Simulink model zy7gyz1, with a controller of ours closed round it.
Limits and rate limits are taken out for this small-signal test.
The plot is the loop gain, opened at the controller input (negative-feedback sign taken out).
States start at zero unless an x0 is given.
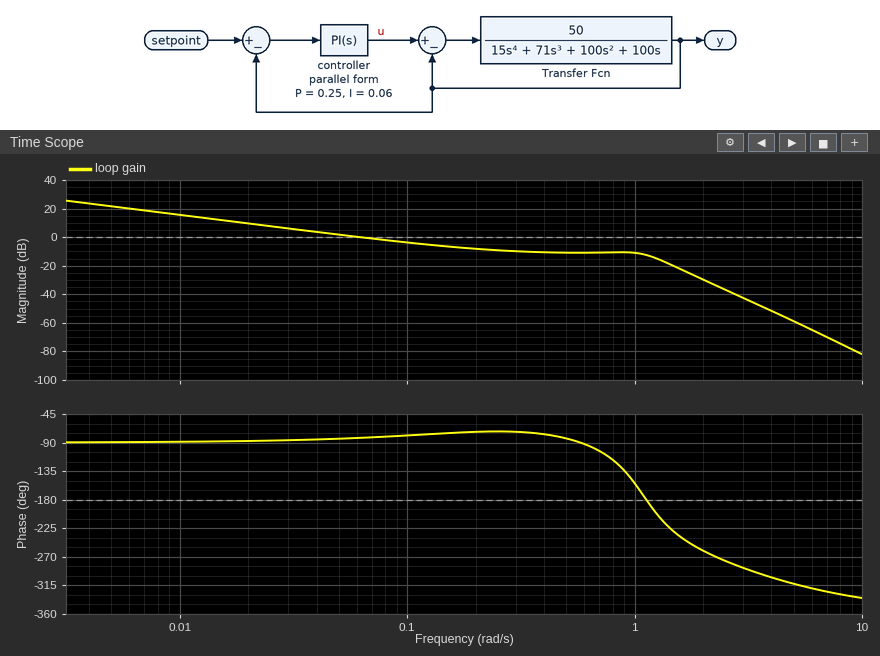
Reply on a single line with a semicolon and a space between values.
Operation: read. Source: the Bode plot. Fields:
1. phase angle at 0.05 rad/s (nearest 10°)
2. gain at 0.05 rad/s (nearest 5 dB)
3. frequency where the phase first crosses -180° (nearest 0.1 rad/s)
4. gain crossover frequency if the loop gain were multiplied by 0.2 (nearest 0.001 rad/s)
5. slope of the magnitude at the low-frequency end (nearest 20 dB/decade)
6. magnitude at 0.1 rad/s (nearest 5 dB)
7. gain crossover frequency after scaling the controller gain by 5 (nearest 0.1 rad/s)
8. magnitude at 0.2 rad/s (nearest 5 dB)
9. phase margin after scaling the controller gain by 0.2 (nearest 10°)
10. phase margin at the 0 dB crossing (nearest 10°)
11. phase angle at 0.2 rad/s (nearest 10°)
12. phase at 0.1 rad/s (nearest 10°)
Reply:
-80°; 0 dB; 1.1 rad/s; 0.012 rad/s; -20 dB/decade; -5 dB; 1.2 rad/s; -10 dB; 90°; 100°; -70°; -80°
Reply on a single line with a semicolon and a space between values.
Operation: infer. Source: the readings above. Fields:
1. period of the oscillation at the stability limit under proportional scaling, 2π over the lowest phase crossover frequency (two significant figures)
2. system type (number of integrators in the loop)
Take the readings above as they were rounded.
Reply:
5.7 s; 1
